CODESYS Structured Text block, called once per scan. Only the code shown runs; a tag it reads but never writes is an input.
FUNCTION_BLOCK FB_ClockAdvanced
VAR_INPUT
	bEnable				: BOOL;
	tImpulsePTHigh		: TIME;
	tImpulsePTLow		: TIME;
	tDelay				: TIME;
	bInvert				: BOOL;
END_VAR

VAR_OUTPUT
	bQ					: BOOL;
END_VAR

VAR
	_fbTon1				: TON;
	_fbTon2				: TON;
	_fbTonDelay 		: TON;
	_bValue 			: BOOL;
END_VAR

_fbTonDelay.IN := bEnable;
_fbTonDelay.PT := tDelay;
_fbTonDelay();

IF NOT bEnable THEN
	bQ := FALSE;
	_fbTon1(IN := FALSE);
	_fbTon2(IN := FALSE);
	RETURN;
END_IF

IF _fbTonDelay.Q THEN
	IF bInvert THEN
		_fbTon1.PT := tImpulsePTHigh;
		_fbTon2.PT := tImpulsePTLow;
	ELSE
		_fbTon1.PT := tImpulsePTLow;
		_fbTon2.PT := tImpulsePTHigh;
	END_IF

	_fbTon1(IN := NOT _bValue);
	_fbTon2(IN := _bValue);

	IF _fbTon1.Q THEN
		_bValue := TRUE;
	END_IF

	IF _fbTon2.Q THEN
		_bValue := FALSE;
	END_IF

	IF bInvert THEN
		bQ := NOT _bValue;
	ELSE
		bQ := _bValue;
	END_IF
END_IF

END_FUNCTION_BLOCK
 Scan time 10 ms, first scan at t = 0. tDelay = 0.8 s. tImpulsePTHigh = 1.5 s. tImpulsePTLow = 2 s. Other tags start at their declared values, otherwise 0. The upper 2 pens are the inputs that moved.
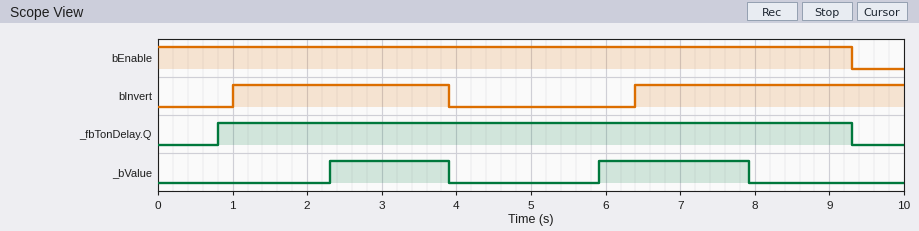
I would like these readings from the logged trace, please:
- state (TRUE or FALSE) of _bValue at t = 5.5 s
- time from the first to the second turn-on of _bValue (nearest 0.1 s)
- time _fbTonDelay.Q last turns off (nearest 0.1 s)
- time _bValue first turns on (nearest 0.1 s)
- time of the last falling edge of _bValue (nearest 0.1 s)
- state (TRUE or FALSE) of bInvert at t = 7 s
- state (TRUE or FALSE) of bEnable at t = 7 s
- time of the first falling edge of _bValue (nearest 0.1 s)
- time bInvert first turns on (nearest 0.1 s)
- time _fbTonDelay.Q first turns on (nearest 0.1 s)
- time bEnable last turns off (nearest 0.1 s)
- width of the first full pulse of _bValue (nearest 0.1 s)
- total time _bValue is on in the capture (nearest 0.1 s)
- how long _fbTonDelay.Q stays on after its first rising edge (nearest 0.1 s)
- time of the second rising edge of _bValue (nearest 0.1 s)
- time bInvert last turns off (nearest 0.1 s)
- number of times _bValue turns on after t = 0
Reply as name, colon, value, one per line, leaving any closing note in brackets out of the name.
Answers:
state (TRUE or FALSE) of _bValue at t = 5.5 s: FALSE
time from the first to the second turn-on of _bValue: 3.6 s
time _fbTonDelay.Q last turns off: 9.3 s
time _bValue first turns on: 2.3 s
time of the last falling edge of _bValue: 7.9 s
state (TRUE or FALSE) of bInvert at t = 7 s: TRUE
state (TRUE or FALSE) of bEnable at t = 7 s: TRUE
time of the first falling edge of _bValue: 3.9 s
time bInvert first turns on: 1.0 s
time _fbTonDelay.Q first turns on: 0.8 s
time bEnable last turns off: 9.3 s
width of the first full pulse of _bValue: 1.6 s
total time _bValue is on in the capture: 3.6 s
how long _fbTonDelay.Q stays on after its first rising edge: 8.5 s
time of the second rising edge of _bValue: 5.9 s
time bInvert last turns off: 3.9 s
number of times _bValue turns on after t = 0: 2
